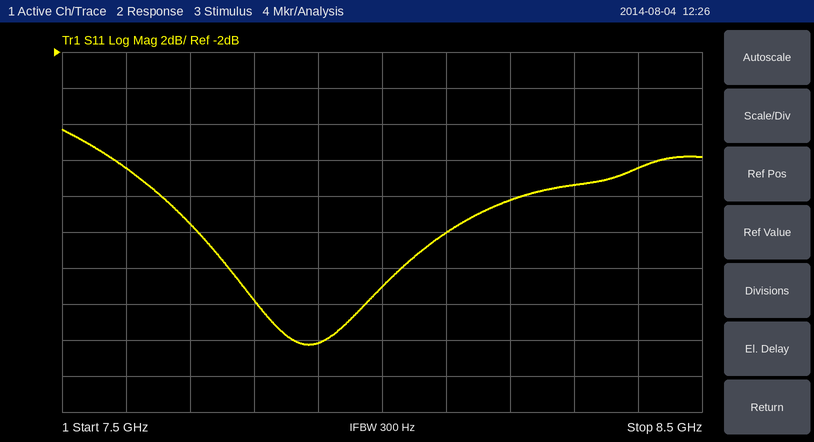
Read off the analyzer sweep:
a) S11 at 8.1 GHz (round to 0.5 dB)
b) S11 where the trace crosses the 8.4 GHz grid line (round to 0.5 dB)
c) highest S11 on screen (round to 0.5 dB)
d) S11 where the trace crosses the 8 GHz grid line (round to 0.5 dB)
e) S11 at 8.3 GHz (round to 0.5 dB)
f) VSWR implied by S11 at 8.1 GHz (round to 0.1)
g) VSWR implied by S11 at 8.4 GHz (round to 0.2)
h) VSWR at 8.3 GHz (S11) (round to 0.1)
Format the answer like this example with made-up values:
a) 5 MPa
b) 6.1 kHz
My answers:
a) -12.0 dB
b) -8.5 dB
c) -6.5 dB
d) -15.0 dB
e) -9.5 dB
f) 1.7
g) 2.2
h) 2.0
